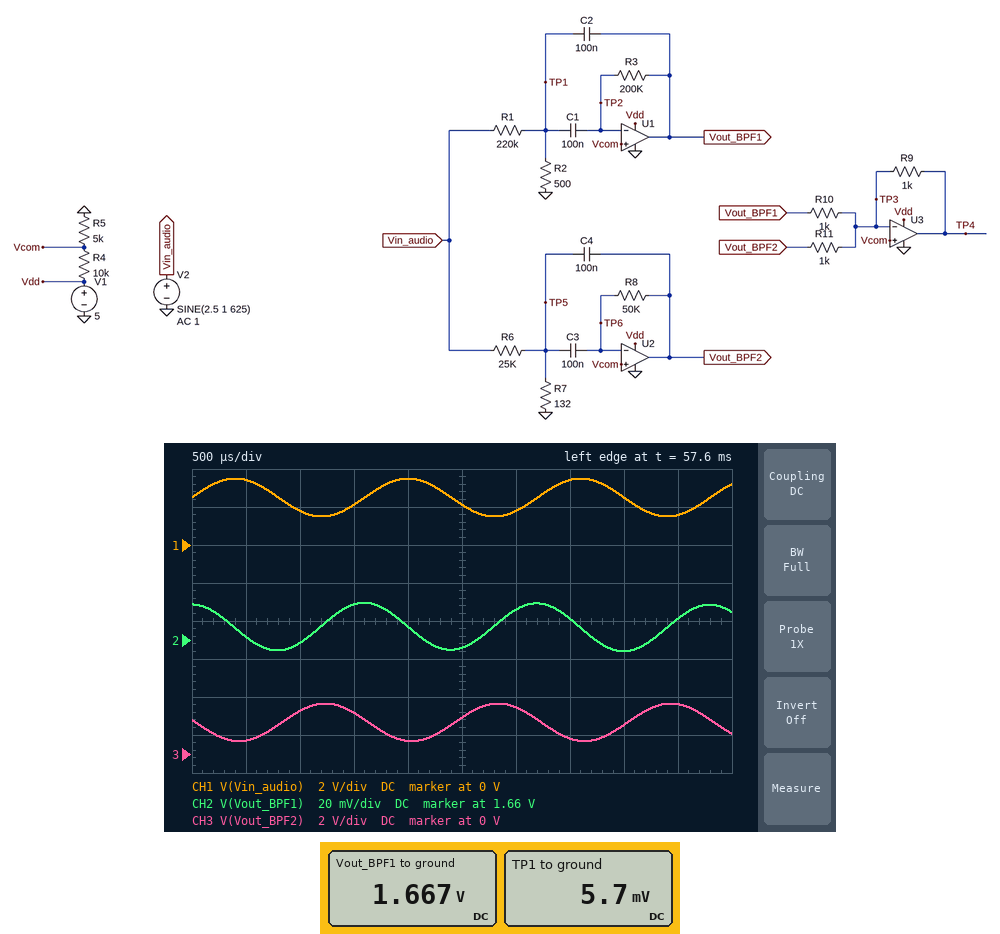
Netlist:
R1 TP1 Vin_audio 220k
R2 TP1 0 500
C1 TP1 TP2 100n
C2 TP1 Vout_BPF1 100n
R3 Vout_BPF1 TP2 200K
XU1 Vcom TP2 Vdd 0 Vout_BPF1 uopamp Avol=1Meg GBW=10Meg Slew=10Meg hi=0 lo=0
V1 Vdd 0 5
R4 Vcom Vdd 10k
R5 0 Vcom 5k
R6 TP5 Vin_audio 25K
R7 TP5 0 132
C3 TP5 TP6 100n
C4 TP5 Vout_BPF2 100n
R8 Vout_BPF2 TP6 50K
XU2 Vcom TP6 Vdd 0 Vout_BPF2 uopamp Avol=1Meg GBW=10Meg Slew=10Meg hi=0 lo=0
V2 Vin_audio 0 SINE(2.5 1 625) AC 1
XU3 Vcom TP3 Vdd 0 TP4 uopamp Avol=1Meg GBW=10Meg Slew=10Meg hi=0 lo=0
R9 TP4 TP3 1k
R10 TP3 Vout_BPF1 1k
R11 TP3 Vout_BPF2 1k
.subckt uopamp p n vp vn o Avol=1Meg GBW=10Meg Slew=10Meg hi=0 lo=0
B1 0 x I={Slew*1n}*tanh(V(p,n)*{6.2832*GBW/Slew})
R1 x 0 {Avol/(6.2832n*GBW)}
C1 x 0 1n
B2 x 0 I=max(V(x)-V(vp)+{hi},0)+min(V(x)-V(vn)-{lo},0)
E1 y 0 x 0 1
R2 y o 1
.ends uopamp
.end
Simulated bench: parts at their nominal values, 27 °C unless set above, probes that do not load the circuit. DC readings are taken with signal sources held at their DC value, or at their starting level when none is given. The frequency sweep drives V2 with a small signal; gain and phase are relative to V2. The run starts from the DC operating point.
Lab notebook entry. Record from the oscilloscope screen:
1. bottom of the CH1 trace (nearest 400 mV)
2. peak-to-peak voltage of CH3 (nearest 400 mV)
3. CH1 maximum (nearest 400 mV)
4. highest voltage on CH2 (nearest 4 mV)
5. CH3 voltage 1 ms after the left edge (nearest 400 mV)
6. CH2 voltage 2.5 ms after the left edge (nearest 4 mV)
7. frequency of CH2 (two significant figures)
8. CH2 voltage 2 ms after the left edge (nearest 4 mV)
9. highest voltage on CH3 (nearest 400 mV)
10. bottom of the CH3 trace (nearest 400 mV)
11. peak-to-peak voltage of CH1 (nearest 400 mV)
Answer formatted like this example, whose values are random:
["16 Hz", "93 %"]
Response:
["1.6 V", "2.0 V", "3.6 V", "1.680 V", "2.4 V", "1.656 V", "620 Hz", "1.668 V", "2.8 V", "800 mV", "2.0 V"]
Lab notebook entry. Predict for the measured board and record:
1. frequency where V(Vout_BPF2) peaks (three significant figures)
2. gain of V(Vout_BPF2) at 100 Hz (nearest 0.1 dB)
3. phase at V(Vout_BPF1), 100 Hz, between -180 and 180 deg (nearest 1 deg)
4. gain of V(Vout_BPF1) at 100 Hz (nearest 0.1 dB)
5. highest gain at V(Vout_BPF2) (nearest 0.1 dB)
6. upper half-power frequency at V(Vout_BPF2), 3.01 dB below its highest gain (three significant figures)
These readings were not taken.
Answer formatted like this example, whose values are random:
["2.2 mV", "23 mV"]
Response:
["621 Hz", "-35.4 dB", "-96 deg", "-26.6 dB", "0 dB", "653 Hz"]
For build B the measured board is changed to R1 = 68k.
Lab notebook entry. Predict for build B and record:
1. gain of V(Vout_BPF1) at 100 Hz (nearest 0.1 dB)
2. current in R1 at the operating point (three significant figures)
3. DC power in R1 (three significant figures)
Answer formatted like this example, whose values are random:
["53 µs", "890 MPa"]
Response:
["-16.5 dB", "36.5 µA", "90.6 µW"]
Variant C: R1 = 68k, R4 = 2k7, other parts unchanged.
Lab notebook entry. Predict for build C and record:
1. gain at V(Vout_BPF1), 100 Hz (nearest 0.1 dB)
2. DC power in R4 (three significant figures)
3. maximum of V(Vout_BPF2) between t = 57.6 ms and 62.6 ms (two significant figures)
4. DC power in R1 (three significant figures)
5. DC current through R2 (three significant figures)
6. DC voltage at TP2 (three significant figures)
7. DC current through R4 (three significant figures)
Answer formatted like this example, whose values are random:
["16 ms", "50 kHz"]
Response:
["-16.5 dB", "1.14 mW", "4.2 V", "90.6 µW", "36.5 µA", "3.25 V", "649 µA"]
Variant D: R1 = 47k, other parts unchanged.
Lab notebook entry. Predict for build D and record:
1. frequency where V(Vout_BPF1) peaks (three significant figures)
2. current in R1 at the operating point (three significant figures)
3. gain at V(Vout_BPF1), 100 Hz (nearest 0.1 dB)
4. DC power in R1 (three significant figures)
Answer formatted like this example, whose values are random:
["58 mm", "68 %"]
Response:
["160 Hz", "52.6 µA", "-13.3 dB", "130 µW"]
